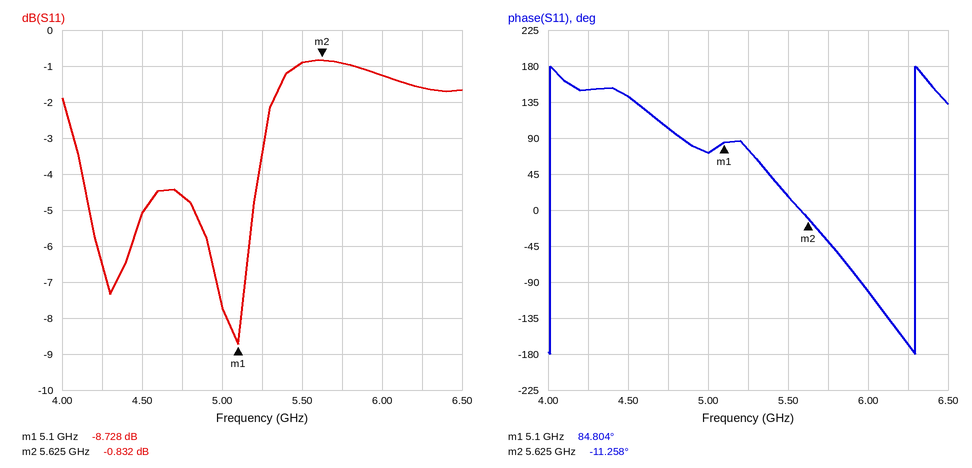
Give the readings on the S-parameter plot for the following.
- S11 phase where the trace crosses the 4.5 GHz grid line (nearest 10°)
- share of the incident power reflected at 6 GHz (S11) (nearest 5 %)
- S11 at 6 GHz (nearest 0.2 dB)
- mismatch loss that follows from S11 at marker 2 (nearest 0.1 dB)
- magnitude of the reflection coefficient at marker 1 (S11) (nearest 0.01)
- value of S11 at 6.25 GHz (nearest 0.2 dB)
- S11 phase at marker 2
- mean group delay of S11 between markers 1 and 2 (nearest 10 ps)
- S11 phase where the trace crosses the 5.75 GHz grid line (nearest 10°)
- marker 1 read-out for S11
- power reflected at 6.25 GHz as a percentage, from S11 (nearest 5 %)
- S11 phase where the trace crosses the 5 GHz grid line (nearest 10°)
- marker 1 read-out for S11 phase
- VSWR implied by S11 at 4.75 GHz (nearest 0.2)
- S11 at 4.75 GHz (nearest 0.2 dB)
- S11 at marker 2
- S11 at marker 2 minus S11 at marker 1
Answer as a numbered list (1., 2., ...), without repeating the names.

1. 140°
2. 75 %
3. -1.2 dB
4. 7.6 dB
5. 0.37
6. -1.6 dB
7. -11.258°
8. 510 ps
9. -40°
10. -8.728 dB
11. 70 %
12. 70°
13. 84.804°
14. 3.8
15. -4.6 dB
16. -0.832 dB
17. 7.896 dB
